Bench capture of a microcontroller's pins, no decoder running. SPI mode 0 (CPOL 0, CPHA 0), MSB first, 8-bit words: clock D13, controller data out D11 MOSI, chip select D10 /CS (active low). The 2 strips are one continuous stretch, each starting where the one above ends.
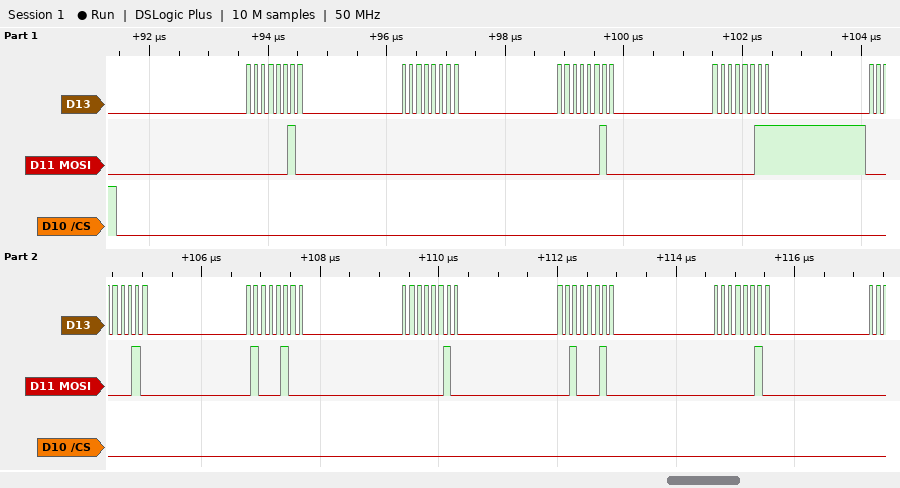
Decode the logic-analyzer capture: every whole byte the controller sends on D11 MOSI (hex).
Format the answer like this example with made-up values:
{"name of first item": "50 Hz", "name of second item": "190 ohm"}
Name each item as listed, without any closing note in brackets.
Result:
{"every whole byte the controller sends on D11 MOSI": "02 00 02 03 02 44 02 22 02"}
